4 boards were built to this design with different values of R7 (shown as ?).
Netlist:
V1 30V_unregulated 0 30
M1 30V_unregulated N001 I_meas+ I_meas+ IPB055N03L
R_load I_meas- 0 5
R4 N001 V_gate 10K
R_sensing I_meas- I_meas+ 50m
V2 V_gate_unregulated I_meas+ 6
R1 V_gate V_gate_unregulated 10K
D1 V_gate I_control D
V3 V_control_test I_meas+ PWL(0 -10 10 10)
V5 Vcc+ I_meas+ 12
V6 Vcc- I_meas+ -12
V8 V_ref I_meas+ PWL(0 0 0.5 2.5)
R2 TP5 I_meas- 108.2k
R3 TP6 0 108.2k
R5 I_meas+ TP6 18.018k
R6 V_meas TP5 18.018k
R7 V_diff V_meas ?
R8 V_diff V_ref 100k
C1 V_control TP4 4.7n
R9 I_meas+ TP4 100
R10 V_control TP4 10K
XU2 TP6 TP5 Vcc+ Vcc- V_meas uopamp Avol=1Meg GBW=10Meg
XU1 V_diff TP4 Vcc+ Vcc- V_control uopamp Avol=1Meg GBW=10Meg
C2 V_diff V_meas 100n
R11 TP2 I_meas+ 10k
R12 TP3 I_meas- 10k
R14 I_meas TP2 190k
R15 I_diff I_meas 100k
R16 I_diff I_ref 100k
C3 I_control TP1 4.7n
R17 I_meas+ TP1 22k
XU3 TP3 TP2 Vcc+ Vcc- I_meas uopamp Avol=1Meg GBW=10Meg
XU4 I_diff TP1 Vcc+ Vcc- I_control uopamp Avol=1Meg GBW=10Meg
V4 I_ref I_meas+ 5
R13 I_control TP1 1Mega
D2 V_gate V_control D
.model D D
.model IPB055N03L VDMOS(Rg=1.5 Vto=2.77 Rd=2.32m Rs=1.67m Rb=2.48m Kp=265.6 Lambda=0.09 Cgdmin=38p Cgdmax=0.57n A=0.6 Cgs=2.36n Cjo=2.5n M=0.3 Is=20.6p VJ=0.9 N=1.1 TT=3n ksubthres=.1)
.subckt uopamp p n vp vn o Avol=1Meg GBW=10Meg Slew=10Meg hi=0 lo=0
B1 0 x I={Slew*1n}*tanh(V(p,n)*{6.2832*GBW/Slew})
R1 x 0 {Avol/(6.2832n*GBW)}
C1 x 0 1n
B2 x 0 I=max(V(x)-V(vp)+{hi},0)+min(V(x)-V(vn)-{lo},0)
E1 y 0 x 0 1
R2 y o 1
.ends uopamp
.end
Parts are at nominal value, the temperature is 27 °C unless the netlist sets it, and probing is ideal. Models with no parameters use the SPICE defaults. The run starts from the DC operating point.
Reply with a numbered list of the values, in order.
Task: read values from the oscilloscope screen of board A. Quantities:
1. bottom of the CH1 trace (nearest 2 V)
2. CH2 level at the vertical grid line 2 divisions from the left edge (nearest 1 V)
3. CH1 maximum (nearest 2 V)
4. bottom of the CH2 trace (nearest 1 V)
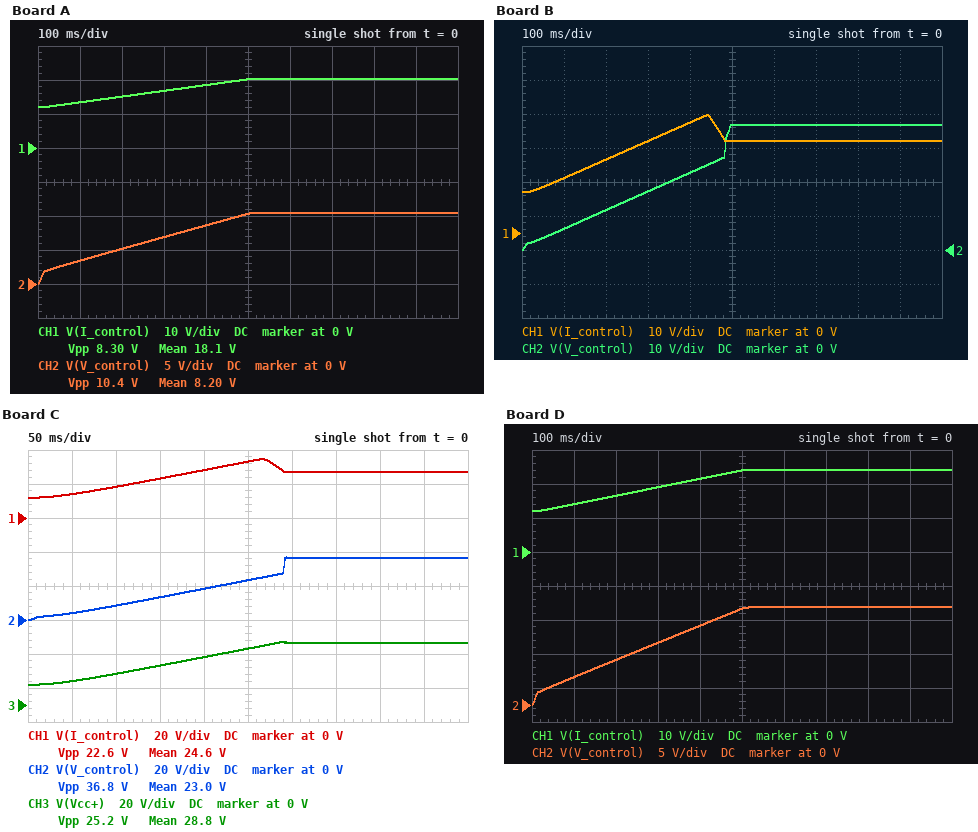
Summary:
1. 12 V
2. 5 V
3. 20 V
4. 0 V
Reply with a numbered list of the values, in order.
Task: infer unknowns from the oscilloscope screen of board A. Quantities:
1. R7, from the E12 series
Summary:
1. 56 kΩ
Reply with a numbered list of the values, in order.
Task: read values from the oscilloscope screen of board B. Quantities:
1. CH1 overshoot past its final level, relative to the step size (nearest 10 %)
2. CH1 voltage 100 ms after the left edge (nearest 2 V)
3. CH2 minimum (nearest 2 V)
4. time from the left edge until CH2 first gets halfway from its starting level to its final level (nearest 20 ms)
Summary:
1. 50 %
2. 16 V
3. 0 V
4. 320 ms
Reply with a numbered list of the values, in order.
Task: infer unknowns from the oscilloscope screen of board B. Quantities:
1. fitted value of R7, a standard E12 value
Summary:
1. 180 kΩ
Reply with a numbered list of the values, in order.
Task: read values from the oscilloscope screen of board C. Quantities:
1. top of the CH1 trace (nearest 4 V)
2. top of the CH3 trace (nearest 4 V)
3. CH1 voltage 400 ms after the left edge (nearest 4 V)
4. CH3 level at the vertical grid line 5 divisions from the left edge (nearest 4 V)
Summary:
1. 36 V
2. 36 V
3. 28 V
4. 32 V
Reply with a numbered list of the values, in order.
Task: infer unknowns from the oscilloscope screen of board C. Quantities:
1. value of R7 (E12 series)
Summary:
1. 330 kΩ
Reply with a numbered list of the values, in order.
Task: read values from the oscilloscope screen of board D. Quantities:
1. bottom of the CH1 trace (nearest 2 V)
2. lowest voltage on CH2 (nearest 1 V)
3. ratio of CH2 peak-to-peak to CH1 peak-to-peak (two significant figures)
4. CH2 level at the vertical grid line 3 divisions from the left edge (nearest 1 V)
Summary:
1. 12 V
2. 0 V
3. 1.2
4. 9 V
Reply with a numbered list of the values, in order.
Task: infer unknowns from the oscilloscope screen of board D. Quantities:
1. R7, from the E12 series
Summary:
1. 82 kΩ
